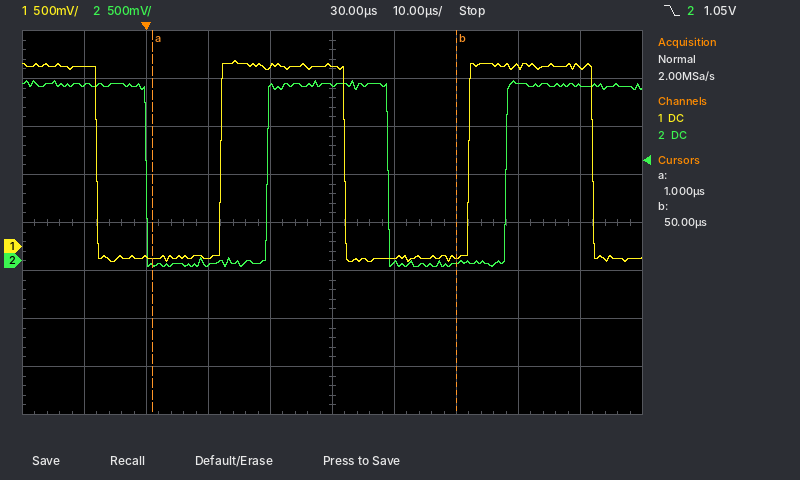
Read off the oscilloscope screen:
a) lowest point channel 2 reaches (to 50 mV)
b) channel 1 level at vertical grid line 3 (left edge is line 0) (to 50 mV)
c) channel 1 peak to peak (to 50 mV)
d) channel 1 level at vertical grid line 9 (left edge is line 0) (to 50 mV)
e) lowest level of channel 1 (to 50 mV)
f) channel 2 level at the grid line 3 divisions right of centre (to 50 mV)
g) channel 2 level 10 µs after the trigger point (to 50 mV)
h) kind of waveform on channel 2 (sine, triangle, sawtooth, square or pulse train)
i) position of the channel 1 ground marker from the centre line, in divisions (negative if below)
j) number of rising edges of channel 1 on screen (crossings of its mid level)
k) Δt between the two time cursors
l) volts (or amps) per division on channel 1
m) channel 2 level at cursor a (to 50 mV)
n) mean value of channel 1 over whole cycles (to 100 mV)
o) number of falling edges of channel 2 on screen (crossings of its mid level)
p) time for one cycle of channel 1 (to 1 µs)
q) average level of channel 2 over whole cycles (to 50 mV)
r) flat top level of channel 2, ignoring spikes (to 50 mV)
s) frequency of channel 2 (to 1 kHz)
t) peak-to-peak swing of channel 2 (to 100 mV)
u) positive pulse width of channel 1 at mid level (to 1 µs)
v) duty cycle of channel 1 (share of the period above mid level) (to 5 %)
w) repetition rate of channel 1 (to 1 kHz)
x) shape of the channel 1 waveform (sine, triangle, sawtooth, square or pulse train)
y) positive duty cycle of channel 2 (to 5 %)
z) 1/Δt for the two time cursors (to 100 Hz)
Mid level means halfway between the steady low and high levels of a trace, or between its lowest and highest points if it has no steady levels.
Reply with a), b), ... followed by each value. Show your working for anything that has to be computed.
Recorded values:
a) -50 mV
b) -100 mV
c) 1.95 V − (-150 mV) = 2.10 V
d) 1.85 V
e) -150 mV
f) 1.85 V
g) -50 mV
h) square
i) -0.5 div
j) 2
k) 50 µs − (1 µs) = 49 µs
l) 500 mV
m) -50 mV
n) -150 mV + 0.5 × (1.95 V − (-150 mV)) ≈ 900 mV
o) 2
p) 40 µs
q) -50 mV + 0.5 × (1.85 V − (-50 mV)) ≈ 900 mV
r) 1.85 V
s) 26 kHz
t) 1.90 V
u) 20 µs
v) 20 µs / 40 µs ≈ 50 %
w) 1 / 40 µs ≈ 25 kHz
x) square
y) 50 %
z) 1 / 49 µs ≈ 20.4 kHz
